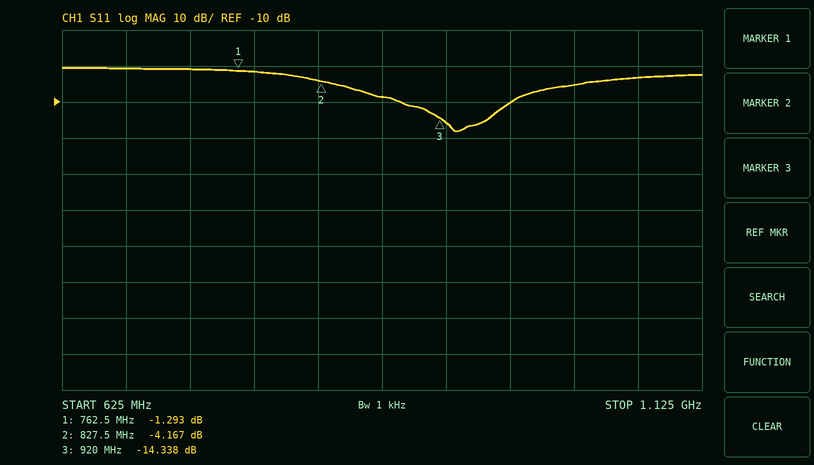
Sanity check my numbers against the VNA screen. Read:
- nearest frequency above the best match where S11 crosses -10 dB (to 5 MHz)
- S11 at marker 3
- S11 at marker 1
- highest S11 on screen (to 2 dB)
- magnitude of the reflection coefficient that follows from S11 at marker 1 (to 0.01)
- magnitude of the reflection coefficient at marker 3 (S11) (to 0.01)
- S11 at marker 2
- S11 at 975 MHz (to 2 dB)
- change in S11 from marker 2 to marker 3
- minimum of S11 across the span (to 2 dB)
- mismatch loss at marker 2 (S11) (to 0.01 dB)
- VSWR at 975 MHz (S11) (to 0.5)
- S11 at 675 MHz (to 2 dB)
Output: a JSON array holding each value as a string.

["975 MHz", "-14.338 dB", "-1.293 dB", "0 dB", "0.86", "0.19", "-4.167 dB", "-10 dB", "-10.171 dB", "-18 dB", "2.10 dB", "2.0", "0 dB"]
